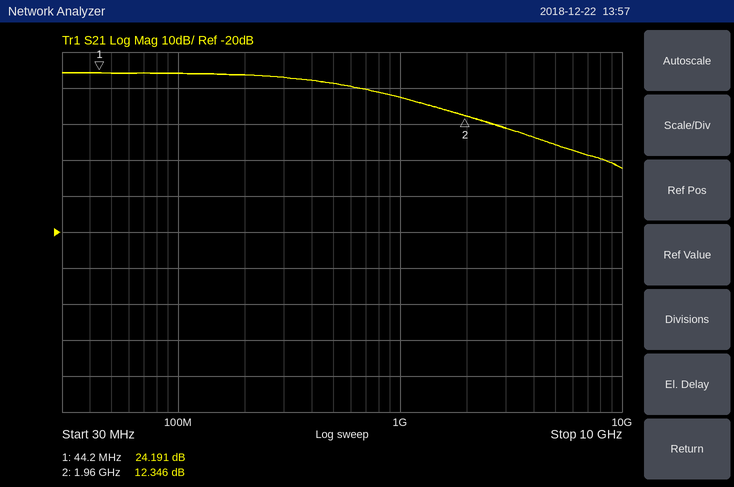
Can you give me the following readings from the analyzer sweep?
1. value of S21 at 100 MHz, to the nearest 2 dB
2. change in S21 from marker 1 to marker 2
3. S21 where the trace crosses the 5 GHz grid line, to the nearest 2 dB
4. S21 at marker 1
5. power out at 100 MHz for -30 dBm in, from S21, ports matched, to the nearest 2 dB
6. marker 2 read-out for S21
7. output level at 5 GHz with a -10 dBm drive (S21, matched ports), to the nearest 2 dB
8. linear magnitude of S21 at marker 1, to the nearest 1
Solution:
24 dB
-11.845 dB
4 dB
24.191 dB
-6 dBm
12.346 dB
-6 dBm
16
